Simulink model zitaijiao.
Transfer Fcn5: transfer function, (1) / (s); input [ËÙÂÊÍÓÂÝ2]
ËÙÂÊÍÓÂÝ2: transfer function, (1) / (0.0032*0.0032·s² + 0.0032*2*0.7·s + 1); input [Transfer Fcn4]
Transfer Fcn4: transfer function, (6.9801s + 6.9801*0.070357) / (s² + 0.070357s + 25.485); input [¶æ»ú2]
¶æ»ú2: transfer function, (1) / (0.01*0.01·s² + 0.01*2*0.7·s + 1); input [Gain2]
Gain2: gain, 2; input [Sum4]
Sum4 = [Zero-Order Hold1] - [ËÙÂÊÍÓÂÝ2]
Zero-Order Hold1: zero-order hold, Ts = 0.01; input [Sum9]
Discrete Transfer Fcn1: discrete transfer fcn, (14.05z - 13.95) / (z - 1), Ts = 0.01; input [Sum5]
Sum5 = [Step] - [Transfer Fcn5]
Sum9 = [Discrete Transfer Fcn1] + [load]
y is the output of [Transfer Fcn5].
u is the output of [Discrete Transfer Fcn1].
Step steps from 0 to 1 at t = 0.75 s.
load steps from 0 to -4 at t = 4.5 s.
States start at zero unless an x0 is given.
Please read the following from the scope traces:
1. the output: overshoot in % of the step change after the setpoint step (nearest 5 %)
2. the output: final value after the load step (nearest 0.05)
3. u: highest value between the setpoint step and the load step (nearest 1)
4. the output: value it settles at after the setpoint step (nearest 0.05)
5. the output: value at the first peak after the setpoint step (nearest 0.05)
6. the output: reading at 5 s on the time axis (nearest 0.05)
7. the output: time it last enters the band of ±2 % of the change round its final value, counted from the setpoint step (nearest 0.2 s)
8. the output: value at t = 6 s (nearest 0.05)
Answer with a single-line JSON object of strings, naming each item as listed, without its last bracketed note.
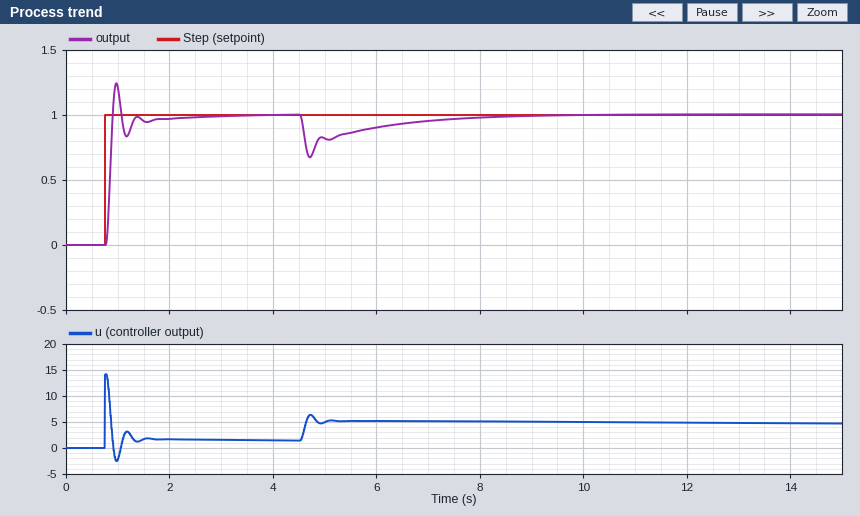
{"the output: overshoot in % of the step change after the setpoint step": "25 %", "the output: final value after the load step": "1.00", "u: highest value between the setpoint step and the load step": "14", "the output: value it settles at after the setpoint step": "1.00", "the output: value at the first peak after the setpoint step": "1.25", "the output: reading at 5 s on the time axis": "0.80", "the output: time it last enters the band of ±2 % of the change round its final value, counted from the setpoint step": "1.6 s", "the output: value at t = 6 s": "0.90"}
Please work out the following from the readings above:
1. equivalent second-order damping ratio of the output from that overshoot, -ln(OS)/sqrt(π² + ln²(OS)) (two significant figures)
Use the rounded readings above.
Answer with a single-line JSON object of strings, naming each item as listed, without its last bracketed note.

{"equivalent second-order damping ratio of the output from that overshoot, -ln(OS)/sqrt(π² + ln²(OS))": "0.40"}
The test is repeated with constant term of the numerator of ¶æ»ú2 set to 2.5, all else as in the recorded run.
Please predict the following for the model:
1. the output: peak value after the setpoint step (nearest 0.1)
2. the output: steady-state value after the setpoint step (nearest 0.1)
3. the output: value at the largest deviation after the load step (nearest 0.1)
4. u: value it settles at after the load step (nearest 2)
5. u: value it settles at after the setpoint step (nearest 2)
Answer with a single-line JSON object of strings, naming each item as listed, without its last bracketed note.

{"the output: peak value after the setpoint step": "1.1", "the output: steady-state value after the setpoint step": "1.0", "the output: value at the largest deviation after the load step": "0.7", "u: value it settles at after the load step": "4", "u: value it settles at after the setpoint step": "0"}
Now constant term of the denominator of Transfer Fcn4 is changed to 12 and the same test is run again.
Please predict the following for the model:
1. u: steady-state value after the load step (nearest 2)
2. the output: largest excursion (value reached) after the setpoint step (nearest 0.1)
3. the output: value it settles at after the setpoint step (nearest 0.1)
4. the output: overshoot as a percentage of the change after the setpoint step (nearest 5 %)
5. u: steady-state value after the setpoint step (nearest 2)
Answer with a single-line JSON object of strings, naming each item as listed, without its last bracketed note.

{"u: steady-state value after the load step": "4", "the output: largest excursion (value reached) after the setpoint step": "1.3", "the output: value it settles at after the setpoint step": "1.0", "the output: overshoot as a percentage of the change after the setpoint step": "30 %", "u: steady-state value after the setpoint step": "0"}
